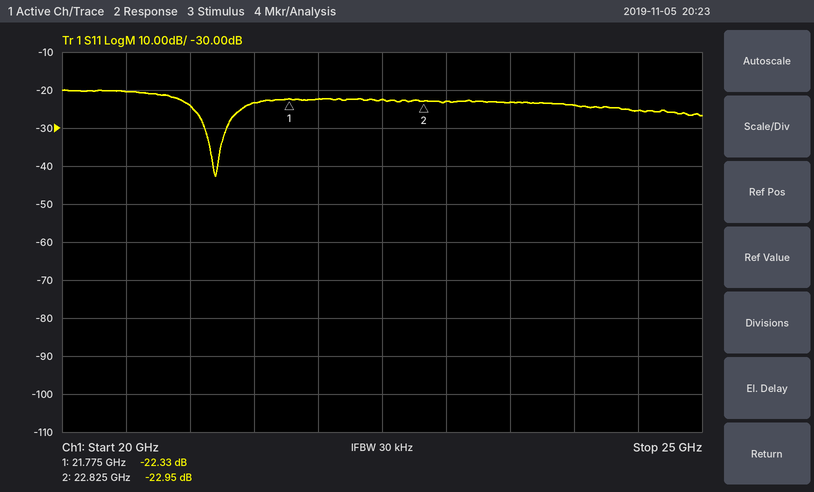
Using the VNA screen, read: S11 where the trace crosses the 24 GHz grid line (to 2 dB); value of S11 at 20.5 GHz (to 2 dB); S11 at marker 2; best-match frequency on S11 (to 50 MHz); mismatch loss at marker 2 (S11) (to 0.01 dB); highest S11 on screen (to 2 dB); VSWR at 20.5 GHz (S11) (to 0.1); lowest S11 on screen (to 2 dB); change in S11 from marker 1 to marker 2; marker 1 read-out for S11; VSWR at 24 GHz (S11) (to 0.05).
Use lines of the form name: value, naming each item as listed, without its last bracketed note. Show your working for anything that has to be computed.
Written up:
S11 where the trace crosses the 24 GHz grid line: -24 dB
value of S11 at 20.5 GHz: -20 dB
S11 at marker 2: -22.95 dB
best-match frequency on S11: 21.20 GHz
mismatch loss at marker 2 (S11): −10 log10(1 − 10^(-22.95/10)) ≈ 0.02 dB
highest S11 on screen: -20 dB
VSWR at 20.5 GHz (S11): |Γ| = 10^(-20/20) = 0.1000; VSWR = (1 + 0.1000)/(1 − 0.1000) ≈ 1.2
lowest S11 on screen: -42 dB
change in S11 from marker 1 to marker 2: -22.95 − (-22.33) = -0.62 dB
marker 1 read-out for S11: -22.33 dB
VSWR at 24 GHz (S11): |Γ| = 10^(-24/20) = 0.0631; VSWR = (1 + 0.0631)/(1 − 0.0631) ≈ 1.13, so 1.15 to the nearest 0.05
